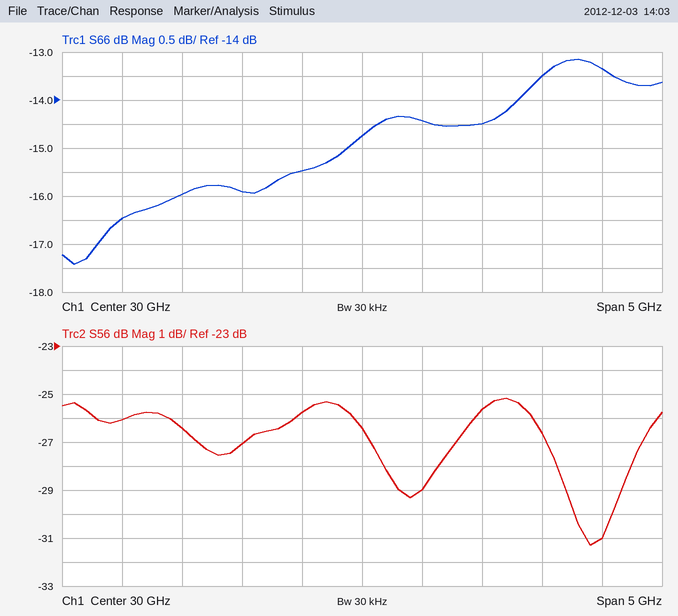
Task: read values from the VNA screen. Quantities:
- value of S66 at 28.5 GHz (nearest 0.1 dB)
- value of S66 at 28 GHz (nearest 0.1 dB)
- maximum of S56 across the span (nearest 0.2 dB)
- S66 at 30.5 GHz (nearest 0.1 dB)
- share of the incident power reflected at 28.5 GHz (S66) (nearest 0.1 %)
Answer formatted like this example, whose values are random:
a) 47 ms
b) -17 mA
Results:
a) -16.0 dB
b) -16.5 dB
c) -25.2 dB
d) -14.4 dB
e) 2.5 %
